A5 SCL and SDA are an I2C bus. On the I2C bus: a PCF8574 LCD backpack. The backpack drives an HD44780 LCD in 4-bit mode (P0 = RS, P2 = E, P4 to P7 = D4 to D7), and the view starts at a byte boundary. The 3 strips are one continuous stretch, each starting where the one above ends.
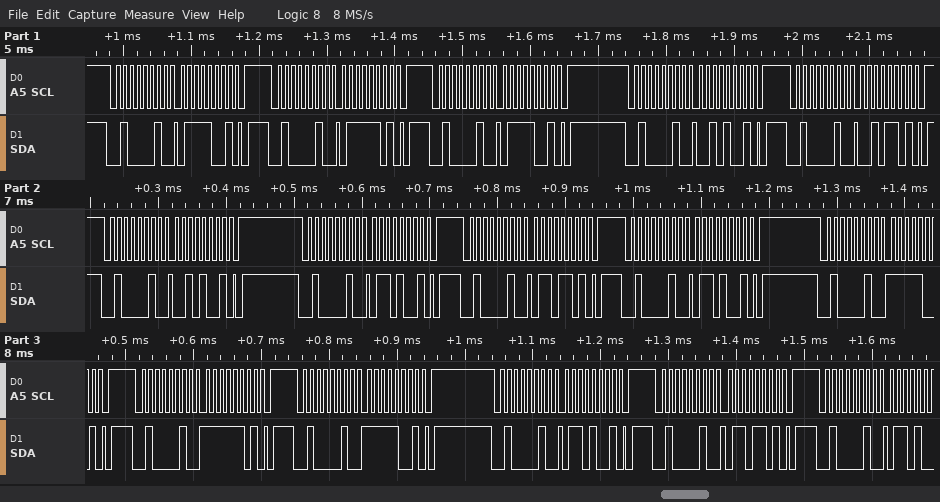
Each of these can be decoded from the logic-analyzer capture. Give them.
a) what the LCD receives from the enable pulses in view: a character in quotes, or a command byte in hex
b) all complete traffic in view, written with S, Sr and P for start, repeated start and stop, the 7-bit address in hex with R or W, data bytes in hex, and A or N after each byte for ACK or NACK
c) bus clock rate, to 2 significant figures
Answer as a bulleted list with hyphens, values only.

- 'r' 'o'
- S 21W A 79 A P S 21W A 7D A P S 21W A 79 A P S 21W A 29 A P S 21W A 2D A P S 21W A 29 A P S 21W A 69 A P S 21W A 6D A P S 21W A 69 A P S 21W A F9 A P S 21W A FD A P S 21W A F9 A P S 21W A 69 A P S 21W A 6D A P S 21W A
- 100 kHz
